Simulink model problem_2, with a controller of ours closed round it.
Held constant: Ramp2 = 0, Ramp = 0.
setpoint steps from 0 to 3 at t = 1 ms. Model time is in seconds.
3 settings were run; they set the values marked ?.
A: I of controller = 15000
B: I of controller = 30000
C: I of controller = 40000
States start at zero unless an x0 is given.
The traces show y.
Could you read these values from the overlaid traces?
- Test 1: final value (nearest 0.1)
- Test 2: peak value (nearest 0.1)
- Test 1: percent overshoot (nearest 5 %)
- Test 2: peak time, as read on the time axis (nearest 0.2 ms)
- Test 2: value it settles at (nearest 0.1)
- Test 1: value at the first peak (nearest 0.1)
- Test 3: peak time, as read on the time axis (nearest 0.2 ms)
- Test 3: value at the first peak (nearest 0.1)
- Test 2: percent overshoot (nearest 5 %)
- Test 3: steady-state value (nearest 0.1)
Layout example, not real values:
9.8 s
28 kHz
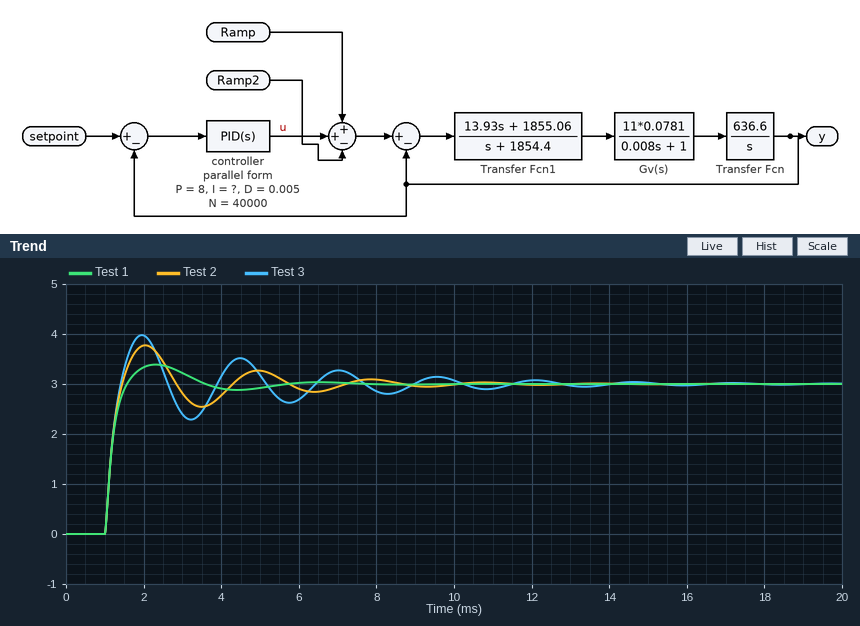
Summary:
3.0
3.8
15 %
2.0 ms
3.0
3.4
2.0 ms
4.0
25 %
3.0
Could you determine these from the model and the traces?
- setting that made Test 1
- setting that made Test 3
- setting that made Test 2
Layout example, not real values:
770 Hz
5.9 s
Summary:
A
C
B
